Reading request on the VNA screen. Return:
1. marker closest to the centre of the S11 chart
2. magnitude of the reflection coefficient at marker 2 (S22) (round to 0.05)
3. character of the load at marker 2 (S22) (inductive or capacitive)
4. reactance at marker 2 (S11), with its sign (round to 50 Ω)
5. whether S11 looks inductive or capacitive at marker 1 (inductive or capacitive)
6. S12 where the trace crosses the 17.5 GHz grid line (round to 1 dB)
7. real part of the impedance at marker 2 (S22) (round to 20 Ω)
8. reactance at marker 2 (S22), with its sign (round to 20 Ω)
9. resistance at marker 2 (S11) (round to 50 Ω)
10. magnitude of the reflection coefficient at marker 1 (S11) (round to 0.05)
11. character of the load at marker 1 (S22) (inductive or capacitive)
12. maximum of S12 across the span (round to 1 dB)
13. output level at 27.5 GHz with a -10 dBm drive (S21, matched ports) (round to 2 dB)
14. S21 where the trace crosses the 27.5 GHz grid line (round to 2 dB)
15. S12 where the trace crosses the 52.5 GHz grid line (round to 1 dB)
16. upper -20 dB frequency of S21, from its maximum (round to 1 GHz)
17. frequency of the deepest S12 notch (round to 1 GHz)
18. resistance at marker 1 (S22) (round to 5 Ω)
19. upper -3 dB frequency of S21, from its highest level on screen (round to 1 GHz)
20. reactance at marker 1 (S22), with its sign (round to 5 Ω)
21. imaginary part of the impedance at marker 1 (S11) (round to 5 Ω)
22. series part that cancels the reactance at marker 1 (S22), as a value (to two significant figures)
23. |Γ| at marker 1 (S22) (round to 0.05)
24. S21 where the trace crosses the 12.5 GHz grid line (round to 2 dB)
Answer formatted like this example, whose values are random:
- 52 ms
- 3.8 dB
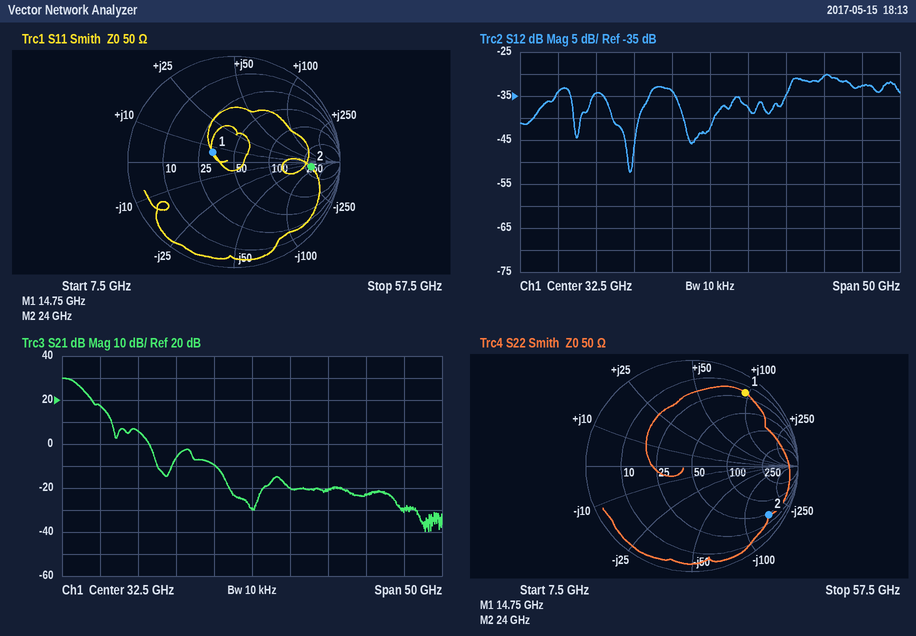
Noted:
- marker 1
- 0.85
- capacitive
- -50 Ω
- inductive
- -34 dB
- 40 Ω
- -160 Ω
- 300 Ω
- 0.20
- inductive
- -30 dB
- -20 dBm
- -10 dB
- -33 dB
- 14 GHz
- 22 GHz
- 20 Ω
- 10 GHz
- +95 Ω
- +5 Ω
- 110 fF
- 0.85
- 18 dB
